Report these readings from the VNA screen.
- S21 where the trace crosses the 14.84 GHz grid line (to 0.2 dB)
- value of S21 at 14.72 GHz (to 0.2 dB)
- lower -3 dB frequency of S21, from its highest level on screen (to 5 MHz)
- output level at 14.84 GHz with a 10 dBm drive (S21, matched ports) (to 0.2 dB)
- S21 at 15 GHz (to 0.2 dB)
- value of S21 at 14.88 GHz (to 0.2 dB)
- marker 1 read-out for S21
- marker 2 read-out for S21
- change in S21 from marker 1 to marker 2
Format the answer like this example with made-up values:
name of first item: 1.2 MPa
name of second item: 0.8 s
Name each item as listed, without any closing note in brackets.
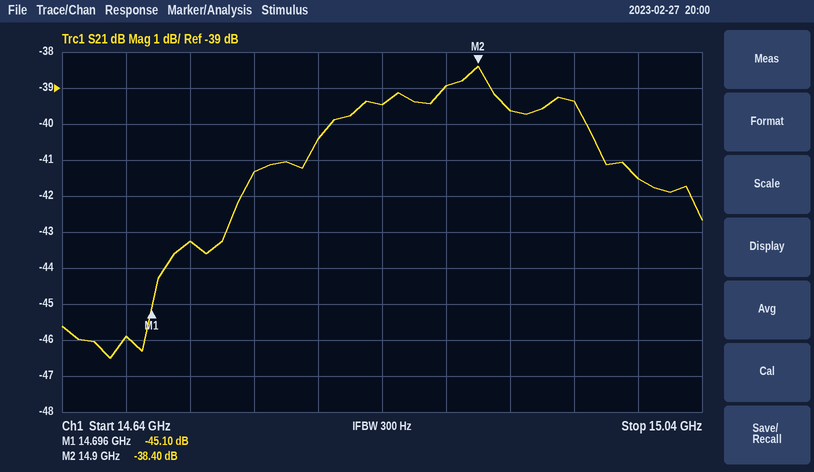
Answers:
S21 where the trace crosses the 14.84 GHz grid line: -39.4 dB
value of S21 at 14.72 GHz: -43.2 dB
lower -3 dB frequency of S21, from its highest level on screen: 14.760 GHz
output level at 14.84 GHz with a 10 dBm drive (S21, matched ports): -29.4 dBm
S21 at 15 GHz: -41.6 dB
value of S21 at 14.88 GHz: -39.0 dB
marker 1 read-out for S21: -45.10 dB
marker 2 read-out for S21: -38.40 dB
change in S21 from marker 1 to marker 2: 6.70 dB
